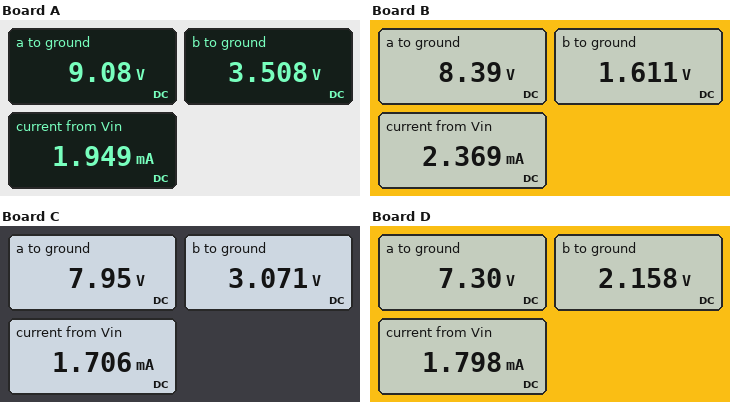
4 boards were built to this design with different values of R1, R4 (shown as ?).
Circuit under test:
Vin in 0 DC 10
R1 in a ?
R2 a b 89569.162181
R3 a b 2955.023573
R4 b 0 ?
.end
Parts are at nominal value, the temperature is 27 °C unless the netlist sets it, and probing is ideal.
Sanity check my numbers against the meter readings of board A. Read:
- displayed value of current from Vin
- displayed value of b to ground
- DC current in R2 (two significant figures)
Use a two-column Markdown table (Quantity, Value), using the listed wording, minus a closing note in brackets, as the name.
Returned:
| Quantity | Value |
|---|---|
| displayed value of current from Vin | 1.949 mA |
| displayed value of b to ground | 3.508 V |
| DC current in R2 | 62 µA |
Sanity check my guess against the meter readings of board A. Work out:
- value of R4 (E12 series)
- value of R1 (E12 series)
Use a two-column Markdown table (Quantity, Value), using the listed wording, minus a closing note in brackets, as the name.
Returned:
| Quantity | Value |
|---|---|
| value of R4 | 1.8 kΩ |
| value of R1 | 470 Ω |
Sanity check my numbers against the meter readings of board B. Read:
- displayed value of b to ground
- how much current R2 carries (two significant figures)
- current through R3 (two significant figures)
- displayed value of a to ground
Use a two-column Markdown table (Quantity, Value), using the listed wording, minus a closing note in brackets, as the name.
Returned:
| Quantity | Value |
|---|---|
| displayed value of b to ground | 1.611 V |
| how much current R2 carries | 76 µA |
| current through R3 | 2.3 mA |
| displayed value of a to ground | 8.39 V |
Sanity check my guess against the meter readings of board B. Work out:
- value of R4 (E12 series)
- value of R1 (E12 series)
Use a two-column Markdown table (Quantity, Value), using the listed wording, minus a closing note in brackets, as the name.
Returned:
| Quantity | Value |
|---|---|
| value of R4 | 680 Ω |
| value of R1 | 680 Ω |
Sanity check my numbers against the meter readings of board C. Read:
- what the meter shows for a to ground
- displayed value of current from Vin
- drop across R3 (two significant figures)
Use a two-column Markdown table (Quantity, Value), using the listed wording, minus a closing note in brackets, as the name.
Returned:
| Quantity | Value |
|---|---|
| what the meter shows for a to ground | 7.95 V |
| displayed value of current from Vin | 1.706 mA |
| drop across R3 | 4.9 V |
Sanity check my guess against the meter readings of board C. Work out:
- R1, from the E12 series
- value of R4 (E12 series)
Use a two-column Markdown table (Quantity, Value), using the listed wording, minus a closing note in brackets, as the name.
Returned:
| Quantity | Value |
|---|---|
| R1, from the E12 series | 1.2 kΩ |
| value of R4 | 1.8 kΩ |
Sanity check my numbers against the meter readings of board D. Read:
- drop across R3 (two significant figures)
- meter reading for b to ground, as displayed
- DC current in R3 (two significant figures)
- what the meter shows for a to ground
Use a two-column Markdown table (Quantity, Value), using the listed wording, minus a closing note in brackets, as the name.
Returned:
| Quantity | Value |
|---|---|
| drop across R3 | 5.1 V |
| meter reading for b to ground, as displayed | 2.158 V |
| DC current in R3 | 1.7 mA |
| what the meter shows for a to ground | 7.30 V |
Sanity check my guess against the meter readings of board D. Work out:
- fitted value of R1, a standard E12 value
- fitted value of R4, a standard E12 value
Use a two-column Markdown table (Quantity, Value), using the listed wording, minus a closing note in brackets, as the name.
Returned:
| Quantity | Value |
|---|---|
| fitted value of R1, a standard E12 value | 1.5 kΩ |
| fitted value of R4, a standard E12 value | 1.2 kΩ |
